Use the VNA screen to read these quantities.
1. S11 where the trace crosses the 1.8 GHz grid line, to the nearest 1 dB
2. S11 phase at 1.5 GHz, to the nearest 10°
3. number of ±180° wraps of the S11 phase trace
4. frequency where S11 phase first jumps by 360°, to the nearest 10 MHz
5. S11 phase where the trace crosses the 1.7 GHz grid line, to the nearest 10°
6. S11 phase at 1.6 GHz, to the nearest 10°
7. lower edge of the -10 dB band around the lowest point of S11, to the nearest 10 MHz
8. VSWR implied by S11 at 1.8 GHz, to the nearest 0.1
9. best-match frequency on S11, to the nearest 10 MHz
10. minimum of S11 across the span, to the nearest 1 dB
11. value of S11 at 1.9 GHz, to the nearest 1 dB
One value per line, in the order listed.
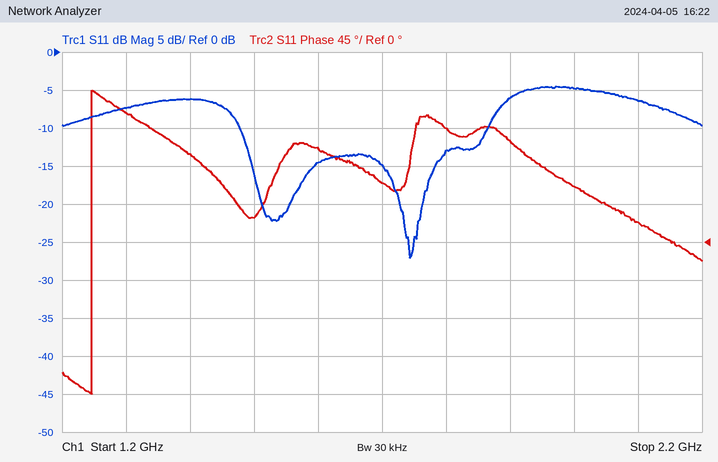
-13 dB
30°
1
1.25 GHz
70°
110°
1.48 GHz
1.6
1.74 GHz
-27 dB
-6 dB
